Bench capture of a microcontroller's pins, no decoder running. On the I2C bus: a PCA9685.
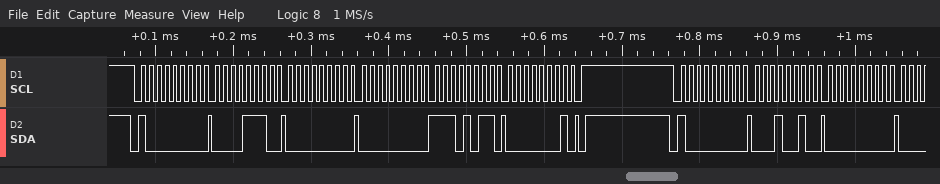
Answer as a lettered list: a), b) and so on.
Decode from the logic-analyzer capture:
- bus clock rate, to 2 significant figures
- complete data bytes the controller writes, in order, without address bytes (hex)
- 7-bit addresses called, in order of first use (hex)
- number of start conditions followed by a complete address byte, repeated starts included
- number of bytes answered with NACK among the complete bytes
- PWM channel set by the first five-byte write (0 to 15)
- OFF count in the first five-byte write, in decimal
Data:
a) 100 kHz
b) 0E 00 00 EB 01 12 00
c) 0x40
d) 2
e) 0
f) 2
g) 491
